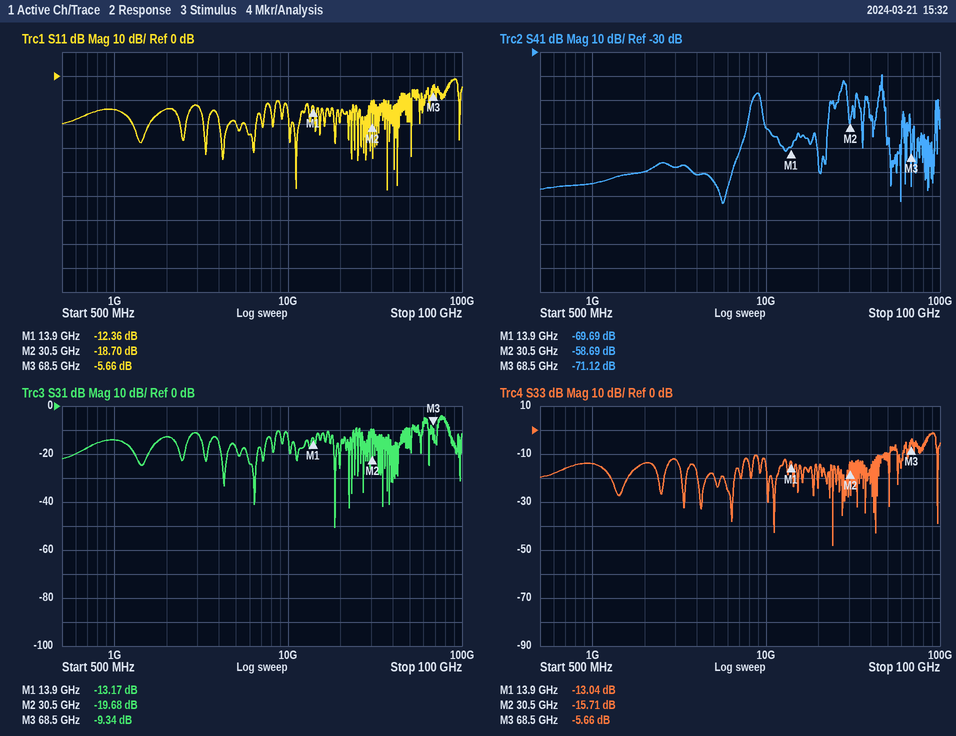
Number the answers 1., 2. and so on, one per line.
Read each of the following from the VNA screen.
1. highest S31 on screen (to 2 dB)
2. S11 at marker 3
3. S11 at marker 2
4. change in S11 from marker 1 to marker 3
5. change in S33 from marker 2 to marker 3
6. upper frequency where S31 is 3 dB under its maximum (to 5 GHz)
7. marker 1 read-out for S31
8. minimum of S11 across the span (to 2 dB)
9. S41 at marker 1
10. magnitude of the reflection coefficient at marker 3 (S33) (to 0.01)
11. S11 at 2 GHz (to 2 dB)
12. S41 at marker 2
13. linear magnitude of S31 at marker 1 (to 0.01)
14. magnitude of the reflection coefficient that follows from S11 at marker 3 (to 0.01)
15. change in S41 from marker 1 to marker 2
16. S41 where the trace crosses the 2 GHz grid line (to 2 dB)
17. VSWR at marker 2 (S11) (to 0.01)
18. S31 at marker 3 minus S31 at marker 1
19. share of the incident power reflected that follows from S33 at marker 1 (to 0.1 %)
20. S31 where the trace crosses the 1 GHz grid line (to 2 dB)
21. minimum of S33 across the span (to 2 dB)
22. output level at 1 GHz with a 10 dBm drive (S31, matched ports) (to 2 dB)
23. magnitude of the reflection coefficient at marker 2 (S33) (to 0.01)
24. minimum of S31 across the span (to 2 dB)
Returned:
1. -4 dB
2. -5.66 dB
3. -18.70 dB
4. 6.70 dB
5. 10.05 dB
6. 80 GHz
7. -13.17 dB
8. -48 dB
9. -69.69 dB
10. 0.52
11. -14 dB
12. -58.69 dB
13. 0.22
14. 0.52
15. 11.00 dB
16. -80 dB
17. 1.26
18. 3.83 dB
19. 5.0 %
20. -14 dB
21. -48 dB
22. -4 dBm
23. 0.16
24. -50 dB
